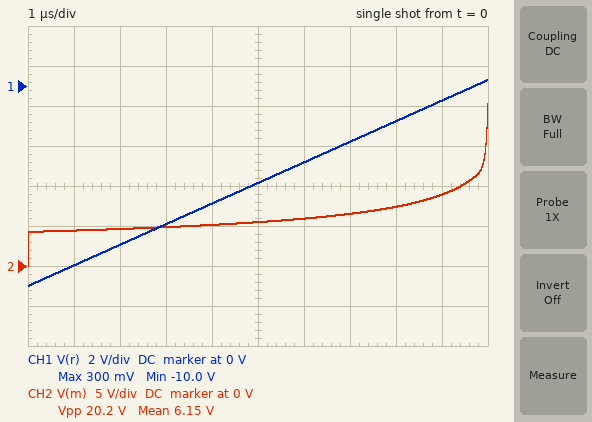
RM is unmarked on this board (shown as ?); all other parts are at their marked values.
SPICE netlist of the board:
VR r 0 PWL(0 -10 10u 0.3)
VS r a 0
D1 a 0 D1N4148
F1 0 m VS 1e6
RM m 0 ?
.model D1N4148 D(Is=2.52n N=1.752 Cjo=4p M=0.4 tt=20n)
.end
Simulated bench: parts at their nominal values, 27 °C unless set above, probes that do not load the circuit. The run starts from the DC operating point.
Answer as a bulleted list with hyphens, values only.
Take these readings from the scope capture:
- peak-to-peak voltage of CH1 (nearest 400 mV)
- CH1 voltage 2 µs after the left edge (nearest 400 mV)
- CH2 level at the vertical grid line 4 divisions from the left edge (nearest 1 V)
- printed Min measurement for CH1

- 10.4 V
- -8.0 V
- 5 V
- -10.0 V
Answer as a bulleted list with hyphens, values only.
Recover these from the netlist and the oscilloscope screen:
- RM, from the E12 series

- 2.7 Ω
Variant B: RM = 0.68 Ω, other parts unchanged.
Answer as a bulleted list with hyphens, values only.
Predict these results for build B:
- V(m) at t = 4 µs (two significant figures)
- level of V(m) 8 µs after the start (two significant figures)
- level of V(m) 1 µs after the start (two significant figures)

- 1.3 V
- 1.9 V
- 1.1 V
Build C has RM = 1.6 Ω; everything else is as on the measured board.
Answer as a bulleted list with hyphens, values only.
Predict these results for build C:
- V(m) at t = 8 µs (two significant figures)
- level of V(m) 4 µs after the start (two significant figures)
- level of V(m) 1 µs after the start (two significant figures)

- 4.4 V
- 3.0 V
- 2.6 V
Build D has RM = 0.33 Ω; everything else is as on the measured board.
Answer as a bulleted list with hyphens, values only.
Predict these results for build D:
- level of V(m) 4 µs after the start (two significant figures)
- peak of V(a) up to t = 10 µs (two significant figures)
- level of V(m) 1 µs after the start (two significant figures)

- 630 mV
- 300 mV
- 540 mV
